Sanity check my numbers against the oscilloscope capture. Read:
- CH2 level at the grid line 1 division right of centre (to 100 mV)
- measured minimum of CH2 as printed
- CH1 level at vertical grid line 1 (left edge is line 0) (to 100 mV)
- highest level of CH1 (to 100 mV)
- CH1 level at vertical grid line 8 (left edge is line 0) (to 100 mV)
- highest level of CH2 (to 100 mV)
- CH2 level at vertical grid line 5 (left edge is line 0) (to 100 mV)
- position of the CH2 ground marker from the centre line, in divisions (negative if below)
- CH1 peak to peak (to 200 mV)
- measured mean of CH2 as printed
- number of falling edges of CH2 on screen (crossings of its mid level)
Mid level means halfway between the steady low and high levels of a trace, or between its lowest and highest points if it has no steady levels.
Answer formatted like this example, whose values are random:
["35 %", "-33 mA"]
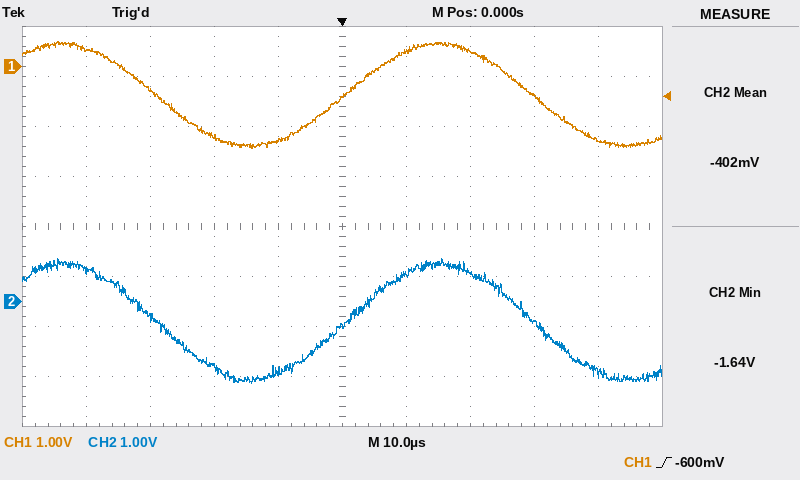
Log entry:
["600 mV", "-1.64 V", "300 mV", "500 mV", "-600 mV", "900 mV", "-500 mV", "-1.5 div", "2.2 V", "-402 mV", "2"]
